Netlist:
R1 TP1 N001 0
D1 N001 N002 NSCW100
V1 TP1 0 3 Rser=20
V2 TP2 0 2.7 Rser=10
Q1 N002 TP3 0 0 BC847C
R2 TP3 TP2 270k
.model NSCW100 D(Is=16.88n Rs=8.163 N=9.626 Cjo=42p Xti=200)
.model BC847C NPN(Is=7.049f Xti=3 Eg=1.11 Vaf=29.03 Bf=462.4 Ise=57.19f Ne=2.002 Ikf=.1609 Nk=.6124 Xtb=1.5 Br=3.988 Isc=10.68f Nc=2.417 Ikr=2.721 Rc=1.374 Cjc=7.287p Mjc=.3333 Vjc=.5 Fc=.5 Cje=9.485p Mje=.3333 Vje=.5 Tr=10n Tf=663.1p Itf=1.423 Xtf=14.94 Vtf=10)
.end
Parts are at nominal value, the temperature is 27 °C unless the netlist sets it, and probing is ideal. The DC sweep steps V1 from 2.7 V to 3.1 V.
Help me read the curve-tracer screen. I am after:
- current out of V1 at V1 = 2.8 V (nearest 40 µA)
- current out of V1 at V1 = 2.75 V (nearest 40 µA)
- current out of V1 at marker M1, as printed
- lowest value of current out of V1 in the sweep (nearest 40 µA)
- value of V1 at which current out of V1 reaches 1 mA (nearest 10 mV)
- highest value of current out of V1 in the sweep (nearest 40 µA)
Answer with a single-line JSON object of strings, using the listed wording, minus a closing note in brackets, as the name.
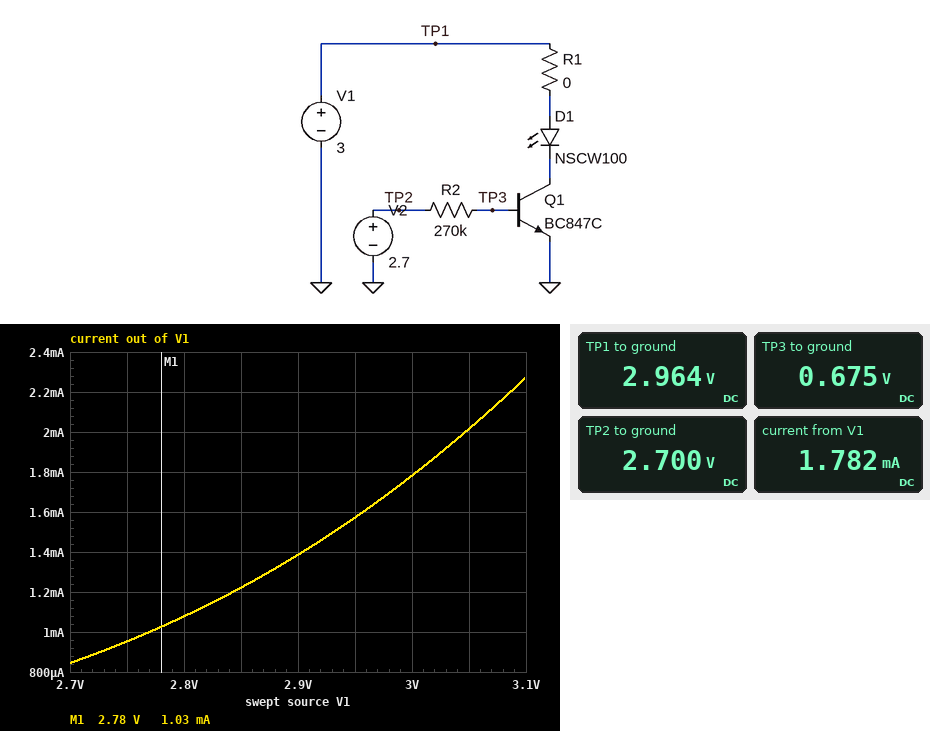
{"current out of V1 at V1 = 2.8 V": "1.08 mA", "current out of V1 at V1 = 2.75 V": "960 µA", "current out of V1 at marker M1, as printed": "1.03 mA", "lowest value of current out of V1 in the sweep": "840 µA", "value of V1 at which current out of V1 reaches 1 mA": "2.77 V", "highest value of current out of V1 in the sweep": "2.28 mA"}
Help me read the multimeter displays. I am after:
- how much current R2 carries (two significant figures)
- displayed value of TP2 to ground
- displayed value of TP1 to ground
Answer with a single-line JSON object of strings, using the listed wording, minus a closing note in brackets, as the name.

{"how much current R2 carries": "7.5 µA", "displayed value of TP2 to ground": "2.700 V", "displayed value of TP1 to ground": "2.964 V"}
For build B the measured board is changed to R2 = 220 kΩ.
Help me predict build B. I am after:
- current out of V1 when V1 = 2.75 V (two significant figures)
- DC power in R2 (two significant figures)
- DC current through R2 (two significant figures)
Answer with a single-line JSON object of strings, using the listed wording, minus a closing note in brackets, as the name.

{"current out of V1 when V1 = 2.75 V": "970 µA", "DC power in R2": "19 µW", "DC current through R2": "9.2 µA"}
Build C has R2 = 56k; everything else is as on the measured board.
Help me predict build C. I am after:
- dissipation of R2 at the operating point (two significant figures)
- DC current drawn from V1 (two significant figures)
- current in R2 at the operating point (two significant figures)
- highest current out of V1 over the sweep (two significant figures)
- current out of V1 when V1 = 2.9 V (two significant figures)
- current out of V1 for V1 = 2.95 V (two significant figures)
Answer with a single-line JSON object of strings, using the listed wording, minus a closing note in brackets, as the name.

{"dissipation of R2 at the operating point": "73 µW", "DC current drawn from V1": "2.0 mA", "current in R2 at the operating point": "36 µA", "highest current out of V1 over the sweep": "2.6 mA", "current out of V1 when V1 = 2.9 V": "1.6 mA", "current out of V1 for V1 = 2.95 V": "1.8 mA"}
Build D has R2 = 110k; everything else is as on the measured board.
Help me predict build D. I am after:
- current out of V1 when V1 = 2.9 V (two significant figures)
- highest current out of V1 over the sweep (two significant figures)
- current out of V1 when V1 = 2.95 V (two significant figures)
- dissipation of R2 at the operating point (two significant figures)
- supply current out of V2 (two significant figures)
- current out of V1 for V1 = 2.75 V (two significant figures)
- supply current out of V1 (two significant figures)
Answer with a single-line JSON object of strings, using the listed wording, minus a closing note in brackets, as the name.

{"current out of V1 when V1 = 2.9 V": "1.5 mA", "highest current out of V1 over the sweep": "2.5 mA", "current out of V1 when V1 = 2.95 V": "1.7 mA", "dissipation of R2 at the operating point": "37 µW", "supply current out of V2": "18 µA", "current out of V1 for V1 = 2.75 V": "1.0 mA", "supply current out of V1": "1.9 mA"}
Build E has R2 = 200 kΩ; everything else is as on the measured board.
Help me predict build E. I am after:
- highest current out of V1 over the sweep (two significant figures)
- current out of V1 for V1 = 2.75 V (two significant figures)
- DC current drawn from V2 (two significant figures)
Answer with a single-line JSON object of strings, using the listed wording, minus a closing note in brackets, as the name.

{"highest current out of V1 over the sweep": "2.4 mA", "current out of V1 for V1 = 2.75 V": "970 µA", "DC current drawn from V2": "10 µA"}
